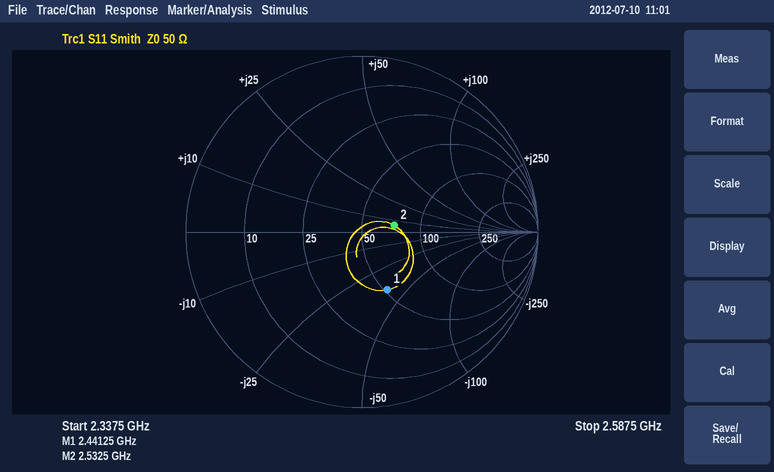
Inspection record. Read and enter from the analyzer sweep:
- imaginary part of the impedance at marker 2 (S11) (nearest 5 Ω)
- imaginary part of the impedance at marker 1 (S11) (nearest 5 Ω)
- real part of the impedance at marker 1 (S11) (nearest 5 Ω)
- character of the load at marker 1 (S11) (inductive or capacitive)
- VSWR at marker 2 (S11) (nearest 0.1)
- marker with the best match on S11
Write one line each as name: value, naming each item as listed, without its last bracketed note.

imaginary part of the impedance at marker 2 (S11): +5 Ω
imaginary part of the impedance at marker 1 (S11): -40 Ω
real part of the impedance at marker 1 (S11): 50 Ω
character of the load at marker 1 (S11): capacitive
VSWR at marker 2 (S11): 1.5
marker with the best match on S11: marker 2
